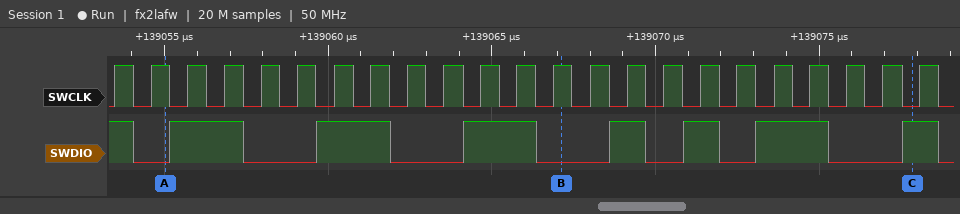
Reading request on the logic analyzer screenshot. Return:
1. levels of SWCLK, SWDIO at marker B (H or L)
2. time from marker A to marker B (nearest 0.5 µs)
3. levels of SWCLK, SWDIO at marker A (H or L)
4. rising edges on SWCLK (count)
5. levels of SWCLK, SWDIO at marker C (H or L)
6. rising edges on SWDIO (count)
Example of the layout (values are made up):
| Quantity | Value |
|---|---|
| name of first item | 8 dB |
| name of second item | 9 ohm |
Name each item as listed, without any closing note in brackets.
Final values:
| Quantity | Value |
|---|---|
| levels of SWCLK, SWDIO at marker B | SWCLK=H, SWDIO=L |
| time from marker A to marker B | 12 µs |
| levels of SWCLK, SWDIO at marker A | SWCLK=H, SWDIO=L |
| rising edges on SWCLK | 23 |
| levels of SWCLK, SWDIO at marker C | SWCLK=L, SWDIO=H |
| rising edges on SWDIO | 7 |
